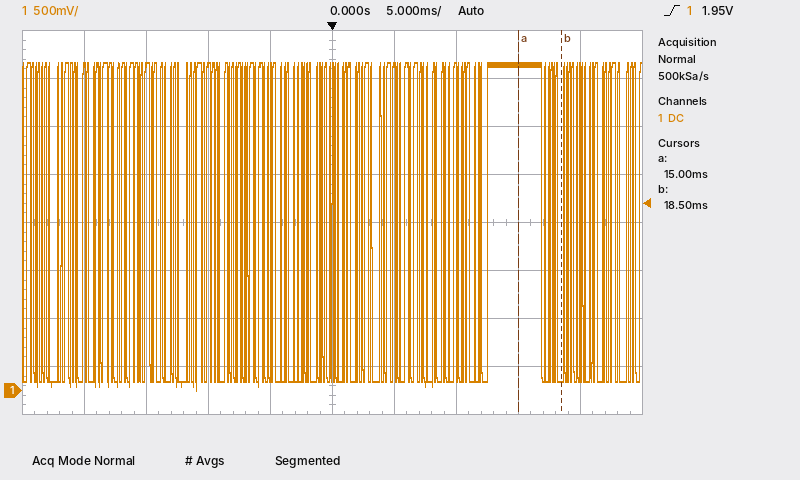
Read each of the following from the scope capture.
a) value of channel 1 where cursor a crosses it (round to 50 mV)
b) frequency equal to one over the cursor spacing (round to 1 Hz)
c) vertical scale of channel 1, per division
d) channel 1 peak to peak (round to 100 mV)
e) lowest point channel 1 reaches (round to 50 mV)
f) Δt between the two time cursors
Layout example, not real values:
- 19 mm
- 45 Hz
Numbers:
- 3.40 V
- 286 Hz
- 500 mV
- 3.40 V
- 0 mV
- 3.5 ms
